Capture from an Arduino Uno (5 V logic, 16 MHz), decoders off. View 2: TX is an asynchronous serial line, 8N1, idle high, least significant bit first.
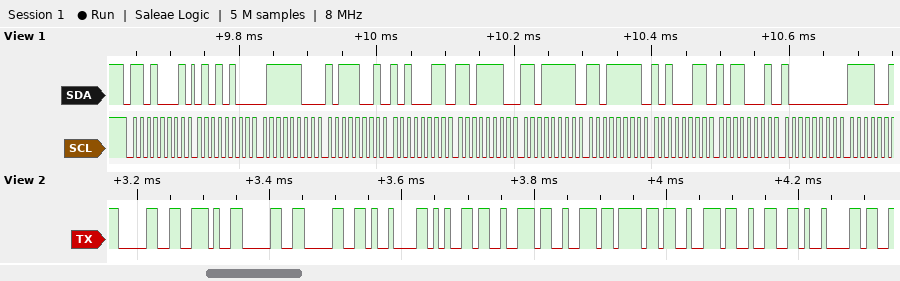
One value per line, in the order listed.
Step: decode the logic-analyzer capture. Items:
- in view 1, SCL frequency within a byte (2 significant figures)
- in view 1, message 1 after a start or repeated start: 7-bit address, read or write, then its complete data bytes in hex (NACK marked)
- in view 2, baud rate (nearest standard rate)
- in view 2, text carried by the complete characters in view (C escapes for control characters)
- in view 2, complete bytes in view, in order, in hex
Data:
100 kHz
0x68 read: 54 7C B9 A3 DE DF DF A3 B1 80
115200 baud
"0.00\terror2\t"
30 2E 30 30 09 65 72 72 6F 72 32 09
